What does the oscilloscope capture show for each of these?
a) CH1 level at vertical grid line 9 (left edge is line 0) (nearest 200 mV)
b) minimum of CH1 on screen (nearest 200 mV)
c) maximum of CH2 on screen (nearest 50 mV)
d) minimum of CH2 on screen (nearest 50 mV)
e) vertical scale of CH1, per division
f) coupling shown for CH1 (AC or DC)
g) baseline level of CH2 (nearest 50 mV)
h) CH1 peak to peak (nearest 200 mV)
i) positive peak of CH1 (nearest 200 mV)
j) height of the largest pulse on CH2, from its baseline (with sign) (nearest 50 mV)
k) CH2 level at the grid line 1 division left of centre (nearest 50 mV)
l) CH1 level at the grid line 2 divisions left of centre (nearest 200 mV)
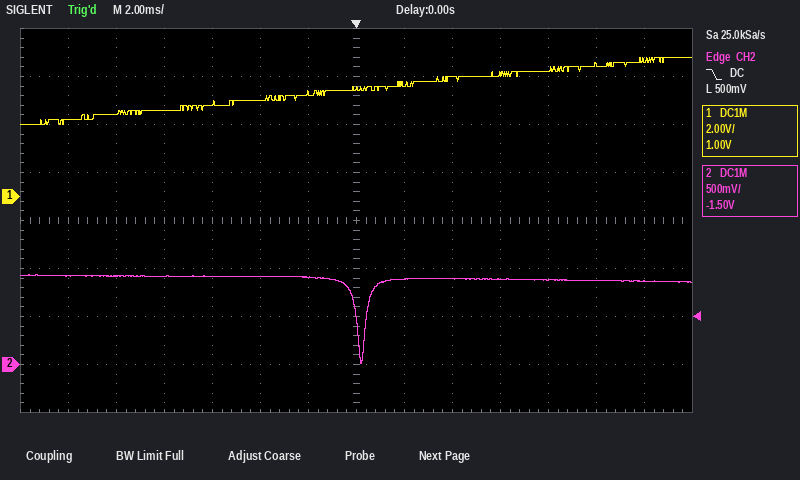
5.0 V
3.0 V
950 mV
0 mV
2 V
DC
900 mV
2.8 V
5.8 V
-900 mV
900 mV
4.0 V
